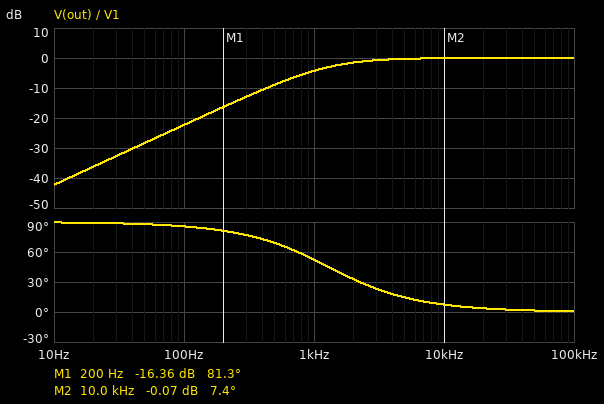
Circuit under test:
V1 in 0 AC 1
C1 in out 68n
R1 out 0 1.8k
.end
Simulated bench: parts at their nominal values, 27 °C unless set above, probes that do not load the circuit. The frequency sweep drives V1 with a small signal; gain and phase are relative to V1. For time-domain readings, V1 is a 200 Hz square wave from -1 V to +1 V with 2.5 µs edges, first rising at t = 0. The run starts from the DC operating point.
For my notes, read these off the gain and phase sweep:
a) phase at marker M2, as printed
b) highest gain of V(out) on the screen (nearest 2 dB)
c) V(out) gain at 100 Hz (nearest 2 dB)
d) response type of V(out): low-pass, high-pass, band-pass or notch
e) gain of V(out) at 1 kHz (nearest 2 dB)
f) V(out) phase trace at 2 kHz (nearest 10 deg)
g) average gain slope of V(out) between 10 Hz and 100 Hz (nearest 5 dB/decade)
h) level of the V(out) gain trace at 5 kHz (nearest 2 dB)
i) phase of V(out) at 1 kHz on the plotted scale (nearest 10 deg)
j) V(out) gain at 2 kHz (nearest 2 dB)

7.4 deg
0 dB
-22 dB
high-pass
-4 dB
30 deg
20 dB/decade
0 dB
50 deg
-2 dB
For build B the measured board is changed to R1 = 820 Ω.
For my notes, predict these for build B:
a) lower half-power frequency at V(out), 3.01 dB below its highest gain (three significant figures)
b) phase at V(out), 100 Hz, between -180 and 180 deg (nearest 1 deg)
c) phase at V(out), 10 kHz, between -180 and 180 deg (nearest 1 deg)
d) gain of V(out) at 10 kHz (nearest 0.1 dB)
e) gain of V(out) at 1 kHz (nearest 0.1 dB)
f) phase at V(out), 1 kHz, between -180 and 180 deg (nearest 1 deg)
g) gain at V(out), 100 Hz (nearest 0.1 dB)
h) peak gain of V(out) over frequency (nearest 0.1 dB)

2.85 kHz
88 deg
16 deg
-0.3 dB
-9.6 dB
71 deg
-29.1 dB
0 dB
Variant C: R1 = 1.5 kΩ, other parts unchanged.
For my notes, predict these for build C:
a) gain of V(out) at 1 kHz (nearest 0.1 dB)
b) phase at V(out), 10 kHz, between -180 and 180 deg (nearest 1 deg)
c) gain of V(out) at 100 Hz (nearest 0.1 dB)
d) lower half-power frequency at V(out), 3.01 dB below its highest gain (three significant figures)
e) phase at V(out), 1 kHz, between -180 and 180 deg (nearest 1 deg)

-5.4 dB
9 deg
-23.9 dB
1.56 kHz
57 deg
